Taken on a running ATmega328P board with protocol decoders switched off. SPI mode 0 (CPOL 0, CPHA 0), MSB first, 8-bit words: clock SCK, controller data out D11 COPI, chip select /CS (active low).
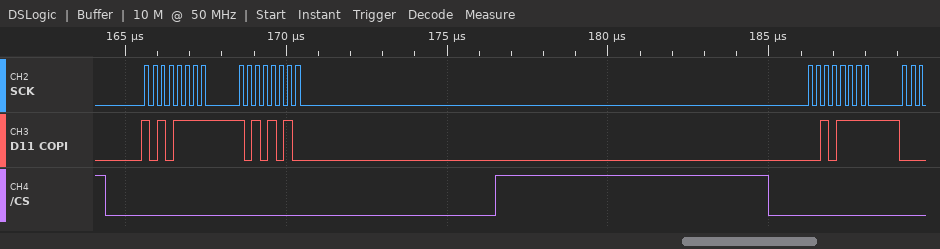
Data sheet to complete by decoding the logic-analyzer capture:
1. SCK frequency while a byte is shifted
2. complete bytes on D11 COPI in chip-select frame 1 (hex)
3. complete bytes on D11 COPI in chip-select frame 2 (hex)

4 MHz
AF AA
2F
